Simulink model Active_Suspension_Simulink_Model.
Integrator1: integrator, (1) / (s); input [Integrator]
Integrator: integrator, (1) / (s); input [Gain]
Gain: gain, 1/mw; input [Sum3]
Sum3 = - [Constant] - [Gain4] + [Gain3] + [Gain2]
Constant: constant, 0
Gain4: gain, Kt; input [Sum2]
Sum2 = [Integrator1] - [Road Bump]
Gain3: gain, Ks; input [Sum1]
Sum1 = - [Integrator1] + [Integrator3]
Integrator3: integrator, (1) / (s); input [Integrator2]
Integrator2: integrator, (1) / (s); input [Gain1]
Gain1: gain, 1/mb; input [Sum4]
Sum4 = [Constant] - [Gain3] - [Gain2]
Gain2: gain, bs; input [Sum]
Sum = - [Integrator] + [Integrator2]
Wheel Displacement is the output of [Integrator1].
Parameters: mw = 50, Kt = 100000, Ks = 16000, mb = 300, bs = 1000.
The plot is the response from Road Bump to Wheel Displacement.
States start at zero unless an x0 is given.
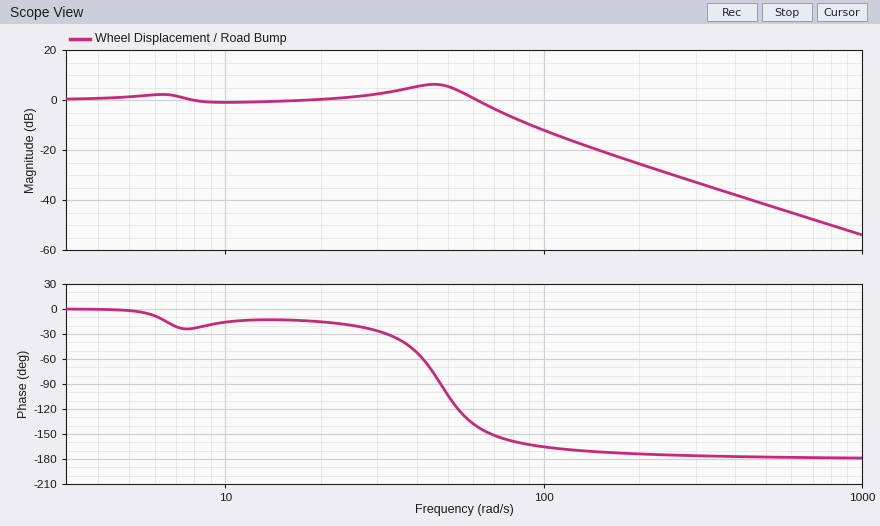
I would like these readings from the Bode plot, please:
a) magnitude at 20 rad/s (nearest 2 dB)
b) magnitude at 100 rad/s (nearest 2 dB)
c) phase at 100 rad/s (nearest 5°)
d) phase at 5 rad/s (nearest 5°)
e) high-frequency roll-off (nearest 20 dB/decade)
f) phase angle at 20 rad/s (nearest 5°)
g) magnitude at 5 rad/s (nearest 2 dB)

0 dB
-12 dB
-165°
0°
-40 dB/decade
-15°
2 dB
